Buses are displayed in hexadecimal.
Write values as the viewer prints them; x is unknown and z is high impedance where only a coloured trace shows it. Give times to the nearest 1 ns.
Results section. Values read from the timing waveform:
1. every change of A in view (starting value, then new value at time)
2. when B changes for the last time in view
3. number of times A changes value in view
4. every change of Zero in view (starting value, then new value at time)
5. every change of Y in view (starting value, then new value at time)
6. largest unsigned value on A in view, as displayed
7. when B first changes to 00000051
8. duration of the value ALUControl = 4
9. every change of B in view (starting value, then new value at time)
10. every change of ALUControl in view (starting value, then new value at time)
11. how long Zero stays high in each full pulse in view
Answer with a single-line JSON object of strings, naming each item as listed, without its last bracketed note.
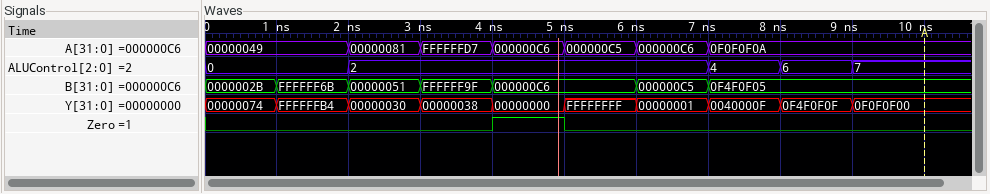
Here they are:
{"every change of A in view": "00000049, 00000081 at 2 ns, FFFFFFD7 at 3 ns, 000000C6 at 4 ns, 000000C5 at 5 ns, 000000C6 at 6 ns, 0F0F0F0A at 7 ns", "when B changes for the last time in view": "7 ns", "number of times A changes value in view": "6", "every change of Zero in view": "0, 1 at 4 ns, 0 at 5 ns", "every change of Y in view": "00000074, FFFFFFB4 at 1 ns, 00000030 at 2 ns, 00000038 at 3 ns, 00000000 at 4 ns, FFFFFFFF at 5 ns, 00000001 at 6 ns, 0040000F at 7 ns, 0F4F0F0F at 8 ns, 0F0F0F00 at 9 ns", "largest unsigned value on A in view, as displayed": "FFFFFFD7", "when B first changes to 00000051": "2 ns", "duration of the value ALUControl = 4": "1 ns", "every change of B in view": "0000002B, FFFFFF6B at 1 ns, 00000051 at 2 ns, FFFFFF9F at 3 ns, 000000C6 at 4 ns, 000000C5 at 6 ns, 0F4F0F05 at 7 ns", "every change of ALUControl in view": "0, 2 at 2 ns, 4 at 7 ns, 6 at 8 ns, 7 at 9 ns", "how long Zero stays high in each full pulse in view": "1 ns"}
